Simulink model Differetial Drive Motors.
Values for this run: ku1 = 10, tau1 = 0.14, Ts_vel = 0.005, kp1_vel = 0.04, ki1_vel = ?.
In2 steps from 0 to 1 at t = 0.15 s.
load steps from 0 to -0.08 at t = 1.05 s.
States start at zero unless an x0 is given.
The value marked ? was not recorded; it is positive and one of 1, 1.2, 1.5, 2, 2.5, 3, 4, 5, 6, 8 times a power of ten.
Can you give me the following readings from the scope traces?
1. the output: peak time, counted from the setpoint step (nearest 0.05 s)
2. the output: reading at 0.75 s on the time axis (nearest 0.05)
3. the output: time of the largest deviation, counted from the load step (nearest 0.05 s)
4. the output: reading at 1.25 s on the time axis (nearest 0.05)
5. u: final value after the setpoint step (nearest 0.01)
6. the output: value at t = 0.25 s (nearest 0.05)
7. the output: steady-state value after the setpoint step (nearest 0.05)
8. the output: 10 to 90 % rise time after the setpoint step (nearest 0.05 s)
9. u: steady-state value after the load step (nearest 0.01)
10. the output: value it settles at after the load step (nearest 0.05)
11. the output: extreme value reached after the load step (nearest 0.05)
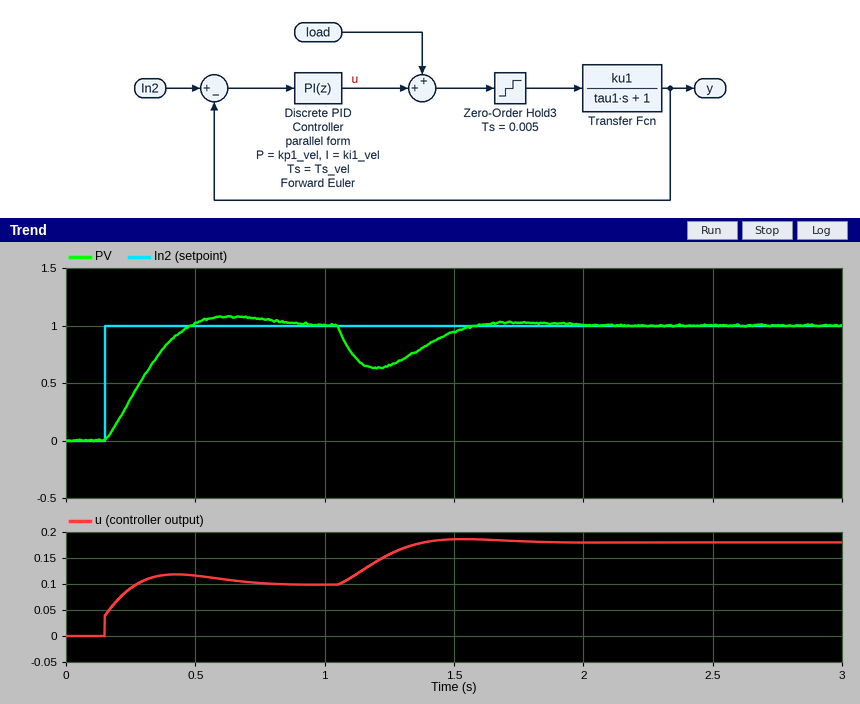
0.50 s
1.05
0.15 s
0.65
0.10
0.35
1.00
0.25 s
0.18
1.00
0.65
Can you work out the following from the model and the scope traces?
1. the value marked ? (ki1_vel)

0.8
